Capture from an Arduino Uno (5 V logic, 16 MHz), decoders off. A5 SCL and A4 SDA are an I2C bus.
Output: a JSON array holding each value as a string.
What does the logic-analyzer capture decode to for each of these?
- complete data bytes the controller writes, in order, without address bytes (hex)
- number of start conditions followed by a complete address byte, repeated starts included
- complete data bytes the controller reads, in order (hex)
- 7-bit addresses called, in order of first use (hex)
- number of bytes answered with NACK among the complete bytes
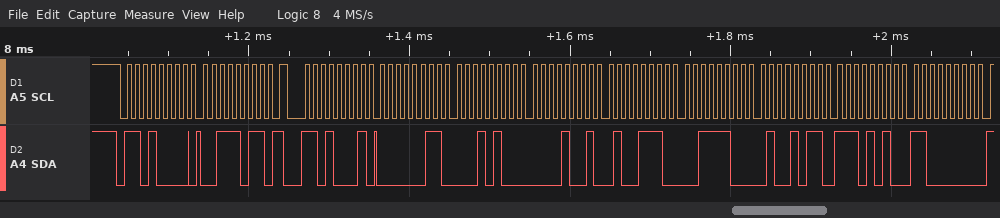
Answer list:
["3B", "2", "03 14 09 4E 3C 4B EA C0", "0x68", "0"]
